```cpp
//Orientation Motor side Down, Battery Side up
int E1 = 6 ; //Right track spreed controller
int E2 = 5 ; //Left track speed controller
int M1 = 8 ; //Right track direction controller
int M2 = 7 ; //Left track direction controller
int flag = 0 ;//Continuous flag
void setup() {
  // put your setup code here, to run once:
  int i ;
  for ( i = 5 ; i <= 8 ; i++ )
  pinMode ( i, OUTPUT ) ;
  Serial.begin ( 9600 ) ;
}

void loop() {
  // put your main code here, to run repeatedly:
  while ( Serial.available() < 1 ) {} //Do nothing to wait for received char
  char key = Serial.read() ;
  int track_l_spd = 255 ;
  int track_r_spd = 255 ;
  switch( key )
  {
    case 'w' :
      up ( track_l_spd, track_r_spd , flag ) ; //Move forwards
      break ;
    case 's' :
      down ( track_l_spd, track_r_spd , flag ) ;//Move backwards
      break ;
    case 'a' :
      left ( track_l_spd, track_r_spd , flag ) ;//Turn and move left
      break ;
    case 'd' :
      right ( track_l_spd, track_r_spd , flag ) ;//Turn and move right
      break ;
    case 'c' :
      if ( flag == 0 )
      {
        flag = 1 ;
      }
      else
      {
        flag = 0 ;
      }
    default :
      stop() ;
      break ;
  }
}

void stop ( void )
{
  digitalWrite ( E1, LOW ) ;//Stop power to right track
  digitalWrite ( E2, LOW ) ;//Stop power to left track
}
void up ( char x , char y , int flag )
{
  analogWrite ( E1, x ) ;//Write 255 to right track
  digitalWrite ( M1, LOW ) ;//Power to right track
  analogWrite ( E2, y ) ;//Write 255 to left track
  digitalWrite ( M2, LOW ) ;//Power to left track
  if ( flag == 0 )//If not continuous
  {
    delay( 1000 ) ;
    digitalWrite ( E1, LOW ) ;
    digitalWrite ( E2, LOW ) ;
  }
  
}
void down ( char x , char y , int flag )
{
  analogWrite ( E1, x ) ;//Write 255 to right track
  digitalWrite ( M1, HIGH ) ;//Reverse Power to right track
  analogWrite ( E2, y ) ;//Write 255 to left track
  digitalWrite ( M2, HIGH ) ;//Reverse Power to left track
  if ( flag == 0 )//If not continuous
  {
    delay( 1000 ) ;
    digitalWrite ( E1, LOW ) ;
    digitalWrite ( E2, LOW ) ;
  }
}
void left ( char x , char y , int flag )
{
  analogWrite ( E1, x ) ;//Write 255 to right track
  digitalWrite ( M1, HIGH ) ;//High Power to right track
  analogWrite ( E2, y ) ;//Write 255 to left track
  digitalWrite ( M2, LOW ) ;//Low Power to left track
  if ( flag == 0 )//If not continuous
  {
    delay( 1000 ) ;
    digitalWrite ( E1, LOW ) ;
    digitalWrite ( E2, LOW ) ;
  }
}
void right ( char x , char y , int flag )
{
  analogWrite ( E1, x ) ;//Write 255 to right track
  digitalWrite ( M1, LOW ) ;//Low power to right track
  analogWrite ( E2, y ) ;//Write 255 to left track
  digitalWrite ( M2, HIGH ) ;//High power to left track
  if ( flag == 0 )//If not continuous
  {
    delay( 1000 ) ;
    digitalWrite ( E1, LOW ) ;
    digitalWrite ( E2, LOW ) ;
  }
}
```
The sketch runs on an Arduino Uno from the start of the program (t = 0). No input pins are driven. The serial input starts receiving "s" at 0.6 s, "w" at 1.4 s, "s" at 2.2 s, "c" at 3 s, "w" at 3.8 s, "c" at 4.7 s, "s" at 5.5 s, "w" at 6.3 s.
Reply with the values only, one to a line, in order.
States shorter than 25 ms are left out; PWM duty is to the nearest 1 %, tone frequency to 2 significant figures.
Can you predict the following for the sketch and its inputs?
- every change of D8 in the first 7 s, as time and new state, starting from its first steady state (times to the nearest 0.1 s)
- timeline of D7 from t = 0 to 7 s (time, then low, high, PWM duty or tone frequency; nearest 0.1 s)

0 s low; 0.6 s high; 1.6 s low; 2.6 s high; 3.8 s low; 5.5 s high; 6.5 s low
0 s low; 0.6 s high; 1.6 s low; 2.6 s high; 3.8 s low; 5.5 s high; 6.5 s low
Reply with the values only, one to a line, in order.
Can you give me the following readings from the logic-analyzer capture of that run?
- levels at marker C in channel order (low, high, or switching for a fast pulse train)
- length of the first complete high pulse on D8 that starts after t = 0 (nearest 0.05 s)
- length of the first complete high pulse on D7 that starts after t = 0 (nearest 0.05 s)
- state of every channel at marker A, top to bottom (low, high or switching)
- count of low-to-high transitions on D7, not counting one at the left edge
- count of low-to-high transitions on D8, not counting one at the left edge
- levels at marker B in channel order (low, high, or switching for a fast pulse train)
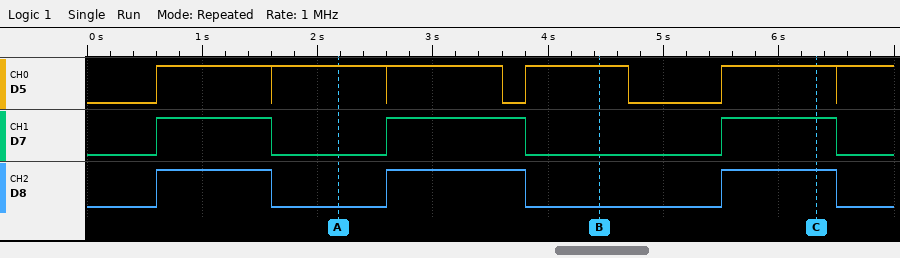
D5 high, D7 high, D8 high
1.00 s
1.00 s
D5 high, D7 low, D8 low
3
3
D5 high, D7 low, D8 low
